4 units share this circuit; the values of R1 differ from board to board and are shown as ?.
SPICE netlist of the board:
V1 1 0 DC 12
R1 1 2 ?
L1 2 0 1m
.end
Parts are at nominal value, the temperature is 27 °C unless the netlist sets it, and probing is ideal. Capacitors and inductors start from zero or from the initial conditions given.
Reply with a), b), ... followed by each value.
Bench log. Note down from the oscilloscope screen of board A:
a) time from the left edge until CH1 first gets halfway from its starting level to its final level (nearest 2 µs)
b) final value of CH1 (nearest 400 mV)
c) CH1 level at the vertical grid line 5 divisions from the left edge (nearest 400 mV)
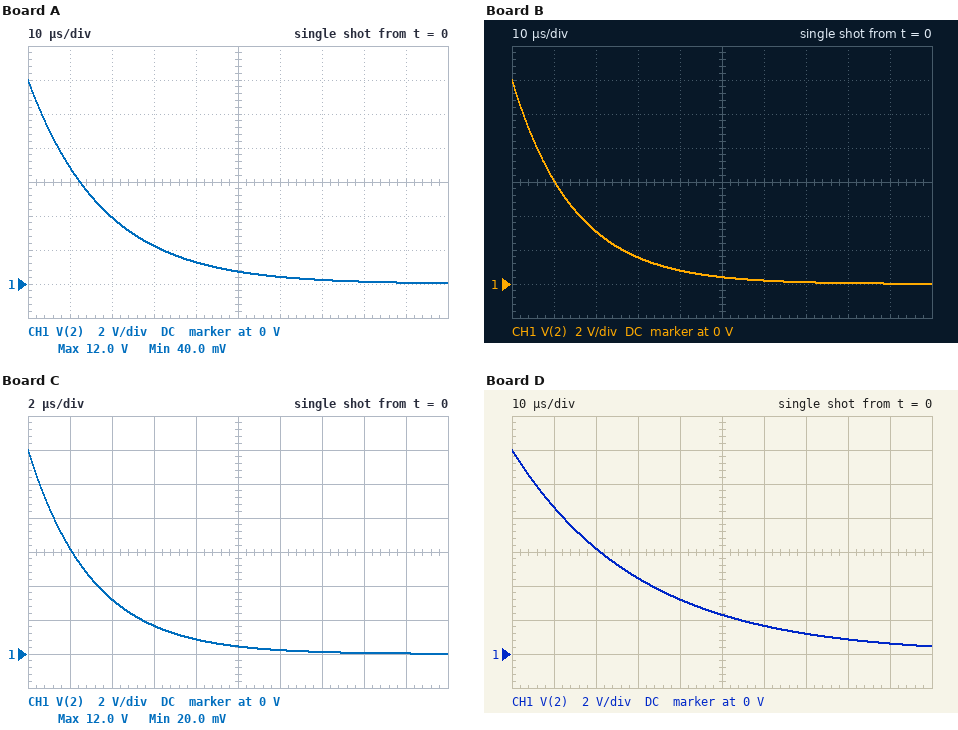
a) 12 µs
b) 0 V
c) 800 mV
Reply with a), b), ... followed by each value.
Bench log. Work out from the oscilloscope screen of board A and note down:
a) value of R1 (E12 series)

a) 56 Ω
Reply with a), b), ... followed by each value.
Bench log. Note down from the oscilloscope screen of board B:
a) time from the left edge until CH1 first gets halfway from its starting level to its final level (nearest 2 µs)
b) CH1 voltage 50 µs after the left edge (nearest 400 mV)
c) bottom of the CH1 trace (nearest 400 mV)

a) 10 µs
b) 400 mV
c) 0 V
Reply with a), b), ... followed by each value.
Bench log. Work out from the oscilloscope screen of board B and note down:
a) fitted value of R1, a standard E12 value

a) 68 Ω
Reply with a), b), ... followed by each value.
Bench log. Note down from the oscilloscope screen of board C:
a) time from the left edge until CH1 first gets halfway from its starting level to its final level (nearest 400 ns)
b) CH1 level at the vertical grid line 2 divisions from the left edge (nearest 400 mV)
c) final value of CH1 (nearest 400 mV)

a) 2.0 µs
b) 3.2 V
c) 0 V
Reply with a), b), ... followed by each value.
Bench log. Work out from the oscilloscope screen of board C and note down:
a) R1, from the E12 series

a) 330 Ω
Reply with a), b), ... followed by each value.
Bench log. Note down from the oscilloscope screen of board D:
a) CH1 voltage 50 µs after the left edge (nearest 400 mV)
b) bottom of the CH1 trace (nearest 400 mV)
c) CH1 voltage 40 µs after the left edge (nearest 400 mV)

a) 2.4 V
b) 400 mV
c) 3.2 V
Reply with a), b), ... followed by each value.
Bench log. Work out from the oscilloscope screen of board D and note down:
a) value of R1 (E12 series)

a) 33 Ω
